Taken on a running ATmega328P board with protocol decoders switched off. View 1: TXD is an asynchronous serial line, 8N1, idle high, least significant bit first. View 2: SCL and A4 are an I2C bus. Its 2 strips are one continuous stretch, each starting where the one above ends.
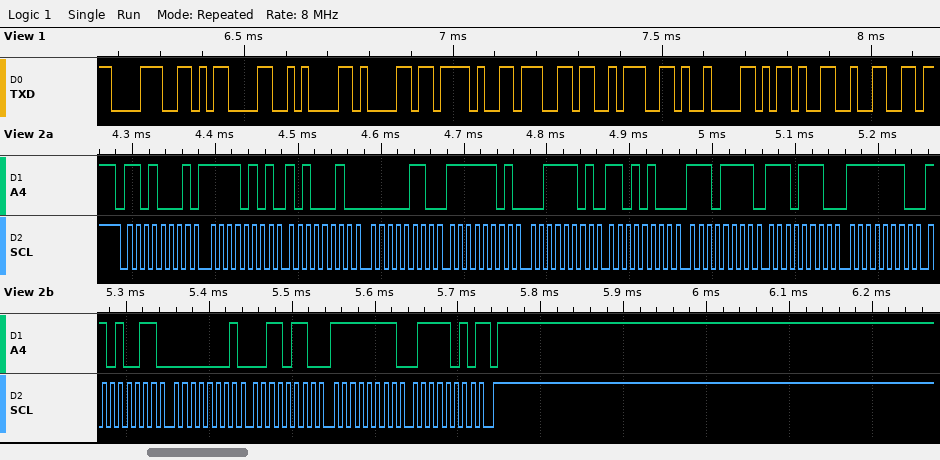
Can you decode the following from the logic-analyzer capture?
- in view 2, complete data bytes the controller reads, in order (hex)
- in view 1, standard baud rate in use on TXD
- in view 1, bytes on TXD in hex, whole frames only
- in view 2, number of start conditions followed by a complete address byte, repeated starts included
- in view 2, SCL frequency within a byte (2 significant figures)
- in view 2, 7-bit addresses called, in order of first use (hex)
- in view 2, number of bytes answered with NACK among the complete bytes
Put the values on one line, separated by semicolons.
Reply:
F5 A2 06 FD 3D D4 EF EE FE D3 01 36 FF 7A; 57600 baud; 38 0D 0A 61 2F 67 3A 09 2D 32; 1; 100 kHz; 0x68; 1
